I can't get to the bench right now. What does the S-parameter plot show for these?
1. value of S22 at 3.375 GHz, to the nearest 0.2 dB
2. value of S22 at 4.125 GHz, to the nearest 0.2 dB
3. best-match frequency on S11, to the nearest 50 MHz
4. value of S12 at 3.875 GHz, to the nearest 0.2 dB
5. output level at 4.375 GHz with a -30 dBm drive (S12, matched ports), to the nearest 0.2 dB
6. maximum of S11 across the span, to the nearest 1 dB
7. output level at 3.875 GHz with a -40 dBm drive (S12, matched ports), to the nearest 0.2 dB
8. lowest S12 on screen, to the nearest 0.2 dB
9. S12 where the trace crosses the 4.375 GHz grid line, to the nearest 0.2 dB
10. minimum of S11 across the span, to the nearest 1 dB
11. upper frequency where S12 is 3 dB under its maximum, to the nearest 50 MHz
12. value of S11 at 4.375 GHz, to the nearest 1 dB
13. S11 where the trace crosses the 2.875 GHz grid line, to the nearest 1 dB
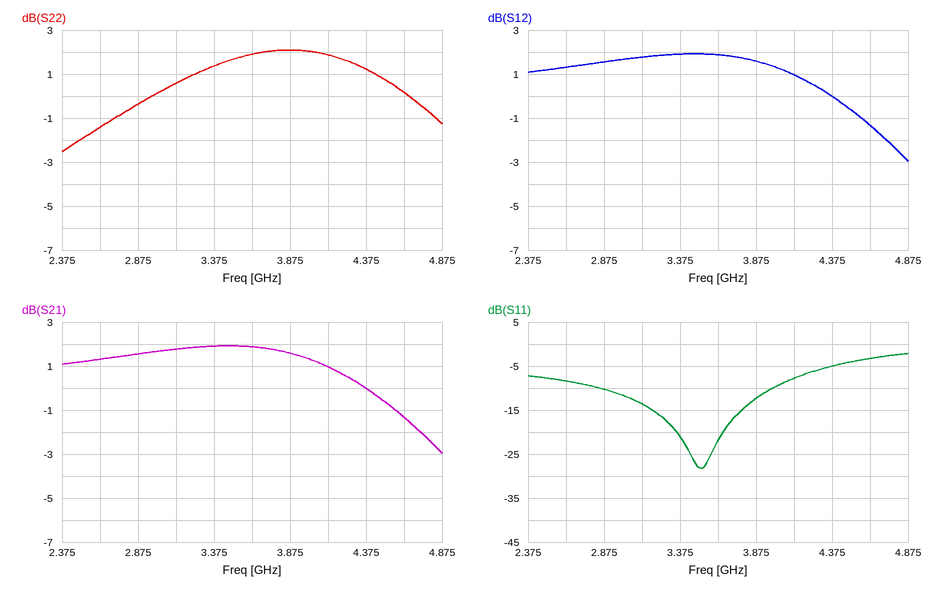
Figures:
1.4 dB
1.8 dB
3.50 GHz
1.6 dB
-30.0 dBm
-2 dB
-38.4 dBm
-3.0 dB
0.0 dB
-28 dB
4.60 GHz
-5 dB
-10 dB
